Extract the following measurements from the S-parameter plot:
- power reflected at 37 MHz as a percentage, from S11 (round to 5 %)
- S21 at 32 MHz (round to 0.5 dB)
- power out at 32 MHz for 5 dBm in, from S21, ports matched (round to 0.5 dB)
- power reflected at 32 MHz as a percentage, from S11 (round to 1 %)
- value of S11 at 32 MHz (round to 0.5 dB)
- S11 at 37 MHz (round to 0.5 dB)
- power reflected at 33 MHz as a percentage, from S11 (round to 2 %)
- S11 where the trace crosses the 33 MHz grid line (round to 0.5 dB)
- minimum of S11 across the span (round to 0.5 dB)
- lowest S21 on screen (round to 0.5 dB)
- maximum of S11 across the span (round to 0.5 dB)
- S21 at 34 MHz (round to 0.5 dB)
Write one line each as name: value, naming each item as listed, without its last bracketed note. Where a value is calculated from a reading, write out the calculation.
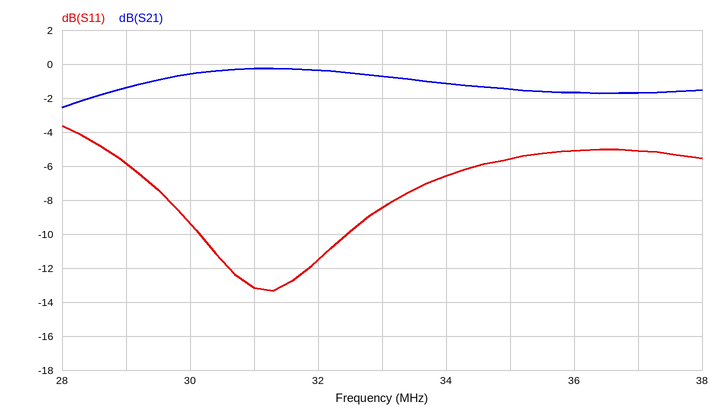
power reflected at 37 MHz as a percentage, from S11: 10^(-5/10) ≈ 31.6 %, so 30 % to the nearest 5 %
S21 at 32 MHz: -0.5 dB
power out at 32 MHz for 5 dBm in, from S21, ports matched: 5 dBm + (-0.5 dB) = 4.5 dBm
power reflected at 32 MHz as a percentage, from S11: 10^(-11.5/10) ≈ 7 %
value of S11 at 32 MHz: -11.5 dB
S11 at 37 MHz: -5.0 dB
power reflected at 33 MHz as a percentage, from S11: 10^(-8.5/10) ≈ 14 %
S11 where the trace crosses the 33 MHz grid line: -8.5 dB
minimum of S11 across the span: -13.5 dB
lowest S21 on screen: -2.5 dB
maximum of S11 across the span: -3.5 dB
S21 at 34 MHz: -1.0 dB
